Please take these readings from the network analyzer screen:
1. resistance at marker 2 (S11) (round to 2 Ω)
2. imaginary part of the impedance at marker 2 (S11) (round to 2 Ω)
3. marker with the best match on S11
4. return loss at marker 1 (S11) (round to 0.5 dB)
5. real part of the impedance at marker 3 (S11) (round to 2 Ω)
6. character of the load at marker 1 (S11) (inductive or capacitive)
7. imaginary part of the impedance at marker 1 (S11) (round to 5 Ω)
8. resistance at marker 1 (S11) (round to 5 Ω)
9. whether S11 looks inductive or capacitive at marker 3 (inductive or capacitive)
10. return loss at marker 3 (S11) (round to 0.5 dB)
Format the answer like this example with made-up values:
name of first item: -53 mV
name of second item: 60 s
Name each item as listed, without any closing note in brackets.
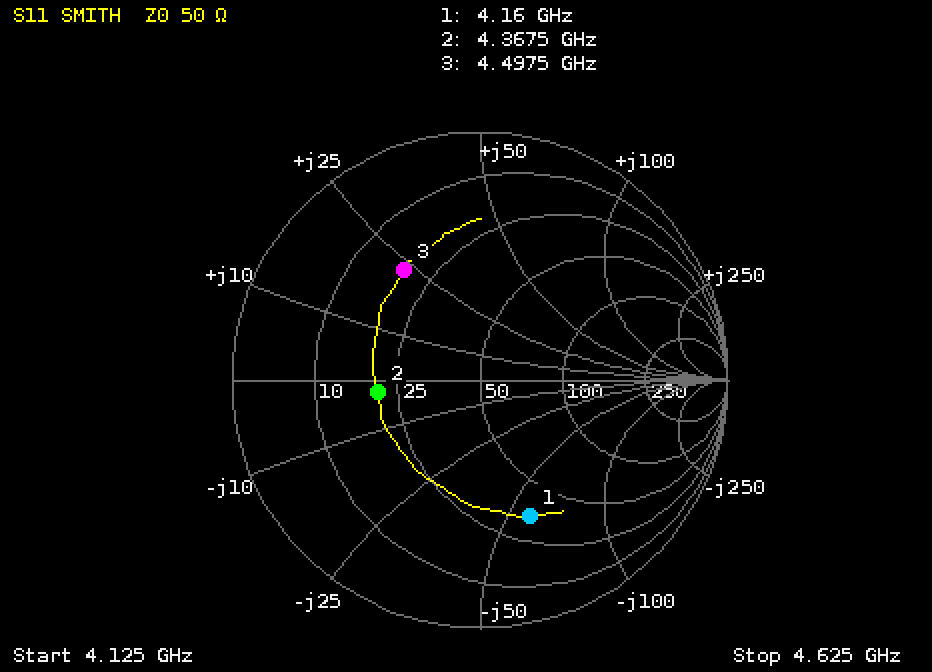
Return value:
resistance at marker 2 (S11): 20 Ω
imaginary part of the impedance at marker 2 (S11): -2 Ω
marker with the best match on S11: marker 2
return loss at marker 1 (S11): 4.5 dB
real part of the impedance at marker 3 (S11): 18 Ω
character of the load at marker 1 (S11): capacitive
imaginary part of the impedance at marker 1 (S11): -60 Ω
resistance at marker 1 (S11): 35 Ω
whether S11 looks inductive or capacitive at marker 3: inductive
return loss at marker 3 (S11): 5.5 dB
